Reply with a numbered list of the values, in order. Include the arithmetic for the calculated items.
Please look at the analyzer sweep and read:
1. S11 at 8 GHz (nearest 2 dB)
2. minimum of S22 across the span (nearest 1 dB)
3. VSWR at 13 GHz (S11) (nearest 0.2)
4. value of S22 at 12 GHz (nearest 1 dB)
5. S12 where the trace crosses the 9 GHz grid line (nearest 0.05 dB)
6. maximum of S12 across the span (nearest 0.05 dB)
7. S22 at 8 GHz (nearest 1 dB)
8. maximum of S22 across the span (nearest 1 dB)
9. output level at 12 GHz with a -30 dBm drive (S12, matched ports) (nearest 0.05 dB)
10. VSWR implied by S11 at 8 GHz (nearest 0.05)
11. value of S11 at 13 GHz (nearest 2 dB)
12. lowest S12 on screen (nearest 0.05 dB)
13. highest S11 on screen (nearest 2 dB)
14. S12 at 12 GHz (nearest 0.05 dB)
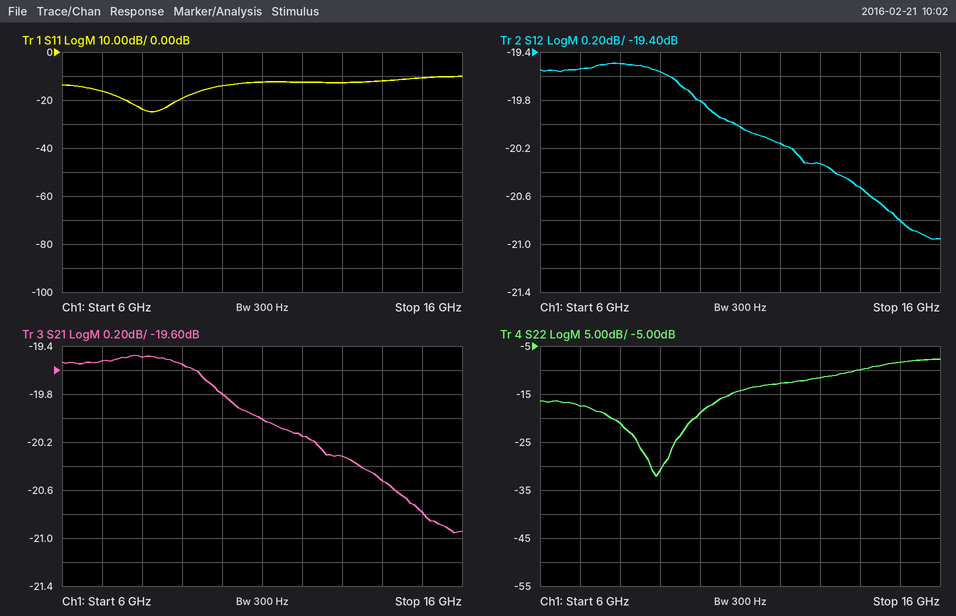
1. -24 dB
2. -32 dB
3. |Γ| = 10^(-12/20) = 0.2512; VSWR = (1 + 0.2512)/(1 − 0.2512) ≈ 1.67, so 1.6 to the nearest 0.2
4. -13 dB
5. -19.55 dB
6. -19.50 dB
7. -21 dB
8. -8 dB
9. -30 dBm + (-20.15 dB) = -50.15 dBm
10. |Γ| = 10^(-24/20) = 0.0631; VSWR = (1 + 0.0631)/(1 − 0.0631) ≈ 1.13, so 1.15 to the nearest 0.05
11. -12 dB
12. -20.95 dB
13. -10 dB
14. -20.15 dB
